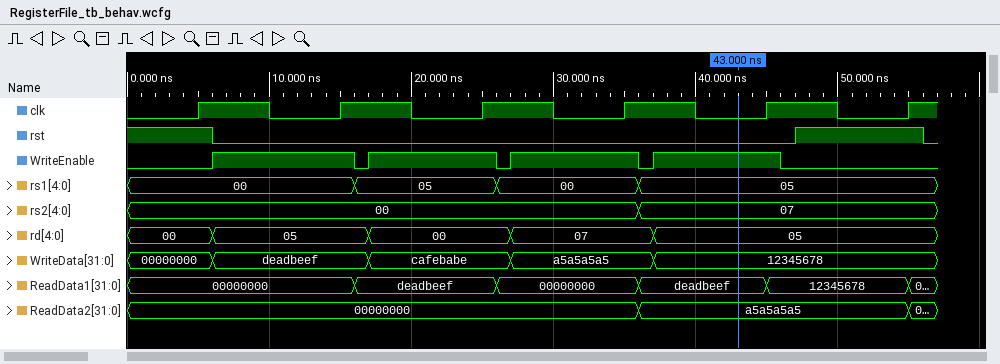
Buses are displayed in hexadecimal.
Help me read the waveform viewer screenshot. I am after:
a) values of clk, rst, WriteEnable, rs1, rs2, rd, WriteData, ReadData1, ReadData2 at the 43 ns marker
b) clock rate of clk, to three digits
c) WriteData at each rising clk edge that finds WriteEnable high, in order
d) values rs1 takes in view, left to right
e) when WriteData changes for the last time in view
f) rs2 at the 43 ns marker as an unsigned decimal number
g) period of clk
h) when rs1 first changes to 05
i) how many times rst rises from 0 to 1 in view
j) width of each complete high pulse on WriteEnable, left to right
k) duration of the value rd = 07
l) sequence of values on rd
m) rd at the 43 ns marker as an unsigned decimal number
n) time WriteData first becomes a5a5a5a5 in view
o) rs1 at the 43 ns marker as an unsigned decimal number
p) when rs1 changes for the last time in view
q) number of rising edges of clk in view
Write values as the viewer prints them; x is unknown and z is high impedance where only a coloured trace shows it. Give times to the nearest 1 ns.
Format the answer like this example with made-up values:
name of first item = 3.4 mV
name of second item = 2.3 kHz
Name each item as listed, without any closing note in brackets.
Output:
values of clk, rst, WriteEnable, rs1, rs2, rd, WriteData, ReadData1, ReadData2 at the 43 ns marker = clk=0, rst=0, WriteEnable=1, rs1=05, rs2=07, rd=05, WriteData=12345678, ReadData1=deadbeef, ReadData2=a5a5a5a5
clock rate of clk, to three digits = 100 MHz
WriteData at each rising clk edge that finds WriteEnable high, in order = deadbeef, cafebabe, a5a5a5a5, 12345678
values rs1 takes in view, left to right = 00, 05, 00, 05
when WriteData changes for the last time in view = 37 ns
rs2 at the 43 ns marker as an unsigned decimal number = 7
period of clk = 10 ns
when rs1 first changes to 05 = 16 ns
how many times rst rises from 0 to 1 in view = 1
width of each complete high pulse on WriteEnable, left to right = 10 ns, 9 ns, 9 ns, 9 ns
duration of the value rd = 07 = 10 ns
sequence of values on rd = 00, 05, 00, 07, 05
rd at the 43 ns marker as an unsigned decimal number = 5
time WriteData first becomes a5a5a5a5 in view = 27 ns
rs1 at the 43 ns marker as an unsigned decimal number = 5
when rs1 changes for the last time in view = 36 ns
number of rising edges of clk in view = 6
